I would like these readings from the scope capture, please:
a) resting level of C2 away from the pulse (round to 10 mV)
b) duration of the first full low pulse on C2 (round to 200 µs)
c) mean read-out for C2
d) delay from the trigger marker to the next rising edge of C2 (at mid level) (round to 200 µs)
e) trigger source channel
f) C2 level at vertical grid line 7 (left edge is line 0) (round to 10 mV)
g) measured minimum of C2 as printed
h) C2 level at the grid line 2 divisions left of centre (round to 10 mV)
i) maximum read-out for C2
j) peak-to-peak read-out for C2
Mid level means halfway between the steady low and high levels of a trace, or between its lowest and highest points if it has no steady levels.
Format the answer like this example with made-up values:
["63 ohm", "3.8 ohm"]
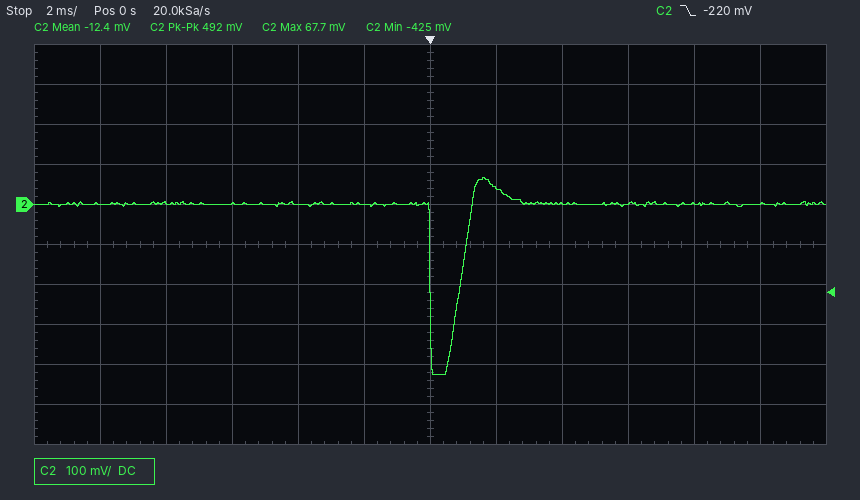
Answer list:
["0 mV", "1.0 ms", "-12.4 mV", "1.0 ms", "C2", "40 mV", "-425 mV", "0 mV", "67.7 mV", "492 mV"]
